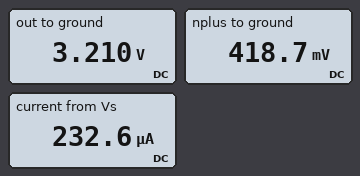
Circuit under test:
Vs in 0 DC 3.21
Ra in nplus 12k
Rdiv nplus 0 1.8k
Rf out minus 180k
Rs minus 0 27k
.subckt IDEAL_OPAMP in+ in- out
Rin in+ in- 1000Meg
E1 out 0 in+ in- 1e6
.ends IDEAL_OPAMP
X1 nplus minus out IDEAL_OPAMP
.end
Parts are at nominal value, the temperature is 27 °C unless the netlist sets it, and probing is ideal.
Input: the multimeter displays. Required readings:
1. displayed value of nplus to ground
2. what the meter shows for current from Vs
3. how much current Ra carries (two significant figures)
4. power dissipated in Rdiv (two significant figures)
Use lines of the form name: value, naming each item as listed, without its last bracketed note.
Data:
displayed value of nplus to ground: 418.7 mV
what the meter shows for current from Vs: 232.6 µA
how much current Ra carries: 230 µA
power dissipated in Rdiv: 97 µW
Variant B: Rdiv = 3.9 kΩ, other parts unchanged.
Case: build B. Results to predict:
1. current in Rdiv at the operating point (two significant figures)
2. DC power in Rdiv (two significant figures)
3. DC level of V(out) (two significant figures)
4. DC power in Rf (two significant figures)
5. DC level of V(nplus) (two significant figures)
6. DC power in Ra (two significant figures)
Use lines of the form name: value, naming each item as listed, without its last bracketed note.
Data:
current in Rdiv at the operating point: 200 µA
DC power in Rdiv: 160 µW
DC level of V(out): 6.0 V
DC power in Rf: 150 µW
DC level of V(nplus): 790 mV
DC power in Ra: 490 µW
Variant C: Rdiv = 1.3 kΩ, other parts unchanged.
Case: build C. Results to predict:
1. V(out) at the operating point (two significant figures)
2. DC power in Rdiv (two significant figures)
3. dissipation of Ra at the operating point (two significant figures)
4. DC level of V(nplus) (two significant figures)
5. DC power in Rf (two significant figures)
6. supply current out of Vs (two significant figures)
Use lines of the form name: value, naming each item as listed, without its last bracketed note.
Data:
V(out) at the operating point: 2.4 V
DC power in Rdiv: 76 µW
dissipation of Ra at the operating point: 700 µW
DC level of V(nplus): 310 mV
DC power in Rf: 24 µW
supply current out of Vs: 240 µA
